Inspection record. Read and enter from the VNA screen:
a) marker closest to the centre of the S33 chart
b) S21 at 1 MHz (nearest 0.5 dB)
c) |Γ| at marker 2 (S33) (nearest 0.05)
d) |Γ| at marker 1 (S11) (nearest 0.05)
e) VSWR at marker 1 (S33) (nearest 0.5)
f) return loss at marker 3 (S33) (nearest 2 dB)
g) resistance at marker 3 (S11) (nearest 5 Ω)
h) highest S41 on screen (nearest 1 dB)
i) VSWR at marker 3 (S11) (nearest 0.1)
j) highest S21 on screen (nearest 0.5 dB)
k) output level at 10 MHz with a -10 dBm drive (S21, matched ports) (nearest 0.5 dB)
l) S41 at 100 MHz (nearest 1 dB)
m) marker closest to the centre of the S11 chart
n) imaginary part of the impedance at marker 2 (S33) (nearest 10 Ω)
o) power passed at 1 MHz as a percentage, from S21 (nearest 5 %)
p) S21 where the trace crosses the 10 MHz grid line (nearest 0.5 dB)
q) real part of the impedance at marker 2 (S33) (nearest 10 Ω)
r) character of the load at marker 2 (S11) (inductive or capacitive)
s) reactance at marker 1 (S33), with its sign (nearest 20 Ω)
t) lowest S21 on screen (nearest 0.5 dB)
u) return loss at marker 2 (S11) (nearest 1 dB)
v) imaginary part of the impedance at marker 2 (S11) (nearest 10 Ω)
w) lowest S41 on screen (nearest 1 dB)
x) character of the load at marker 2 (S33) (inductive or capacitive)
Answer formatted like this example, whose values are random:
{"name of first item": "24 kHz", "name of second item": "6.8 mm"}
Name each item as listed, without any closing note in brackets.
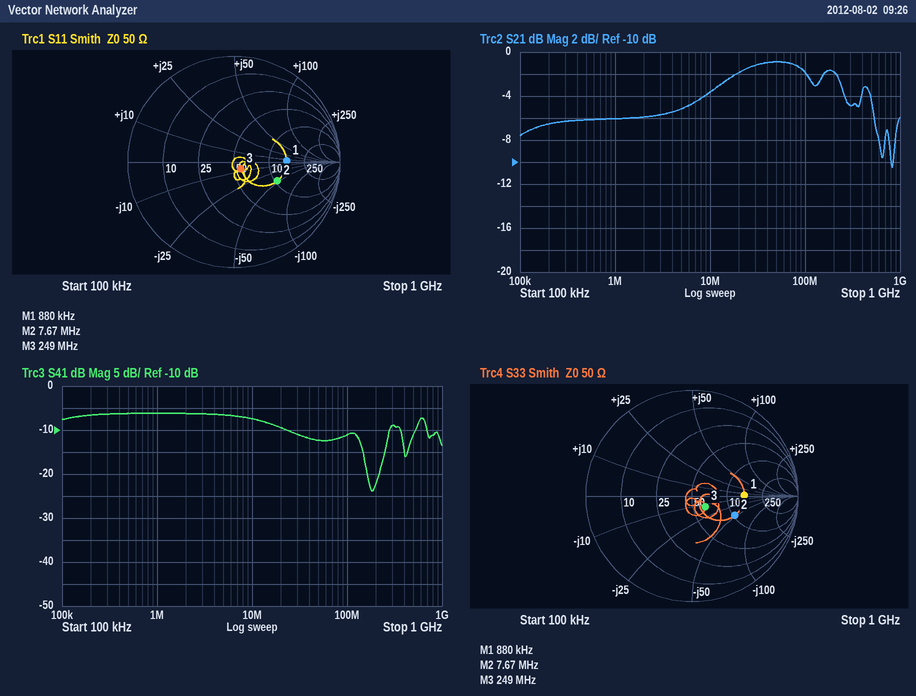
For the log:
{"marker closest to the centre of the S33 chart": "marker 3", "S21 at 1 MHz": "-6.0 dB", "|Γ| at marker 2 (S33)": "0.45", "|Γ| at marker 1 (S11)": "0.50", "VSWR at marker 1 (S33)": "3.0", "return loss at marker 3 (S33)": "16 dB", "resistance at marker 3 (S11)": "55 Ω", "highest S41 on screen": "-6 dB", "VSWR at marker 3 (S11)": "1.2", "highest S21 on screen": "-1.0 dB", "output level at 10 MHz with a -10 dBm drive (S21, matched ports)": "-13.5 dBm", "S41 at 100 MHz": "-11 dB", "marker closest to the centre of the S11 chart": "marker 3", "imaginary part of the impedance at marker 2 (S33)": "-50 Ω", "power passed at 1 MHz as a percentage, from S21": "25 %", "S21 where the trace crosses the 10 MHz grid line": "-3.5 dB", "real part of the impedance at marker 2 (S33)": "100 Ω", "character of the load at marker 2 (S11)": "capacitive", "reactance at marker 1 (S33), with its sign": "0 Ω", "lowest S21 on screen": "-10.5 dB", "return loss at marker 2 (S11)": "7 dB", "imaginary part of the impedance at marker 2 (S11)": "-50 Ω", "lowest S41 on screen": "-24 dB", "character of the load at marker 2 (S33)": "capacitive"}
